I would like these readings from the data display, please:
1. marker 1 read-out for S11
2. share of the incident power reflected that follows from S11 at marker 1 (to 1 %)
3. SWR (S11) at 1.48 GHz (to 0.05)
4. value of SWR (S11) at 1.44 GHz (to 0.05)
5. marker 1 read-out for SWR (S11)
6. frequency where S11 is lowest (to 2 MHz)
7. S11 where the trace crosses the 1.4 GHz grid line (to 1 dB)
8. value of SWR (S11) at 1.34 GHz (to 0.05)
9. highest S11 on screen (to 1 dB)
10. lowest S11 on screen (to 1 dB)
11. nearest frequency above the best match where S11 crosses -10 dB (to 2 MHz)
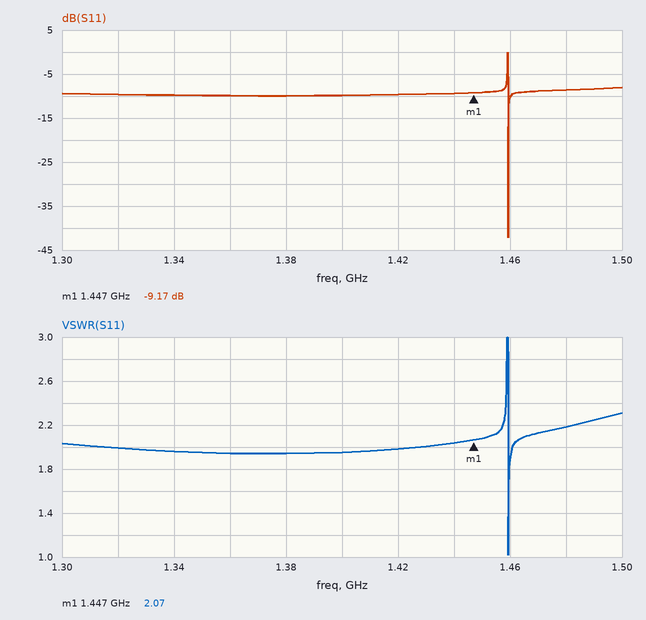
-9.17 dB
12 %
2.20
2.05
2.07
1.460 GHz
-10 dB
1.95
0 dB
-42 dB
1.460 GHz
